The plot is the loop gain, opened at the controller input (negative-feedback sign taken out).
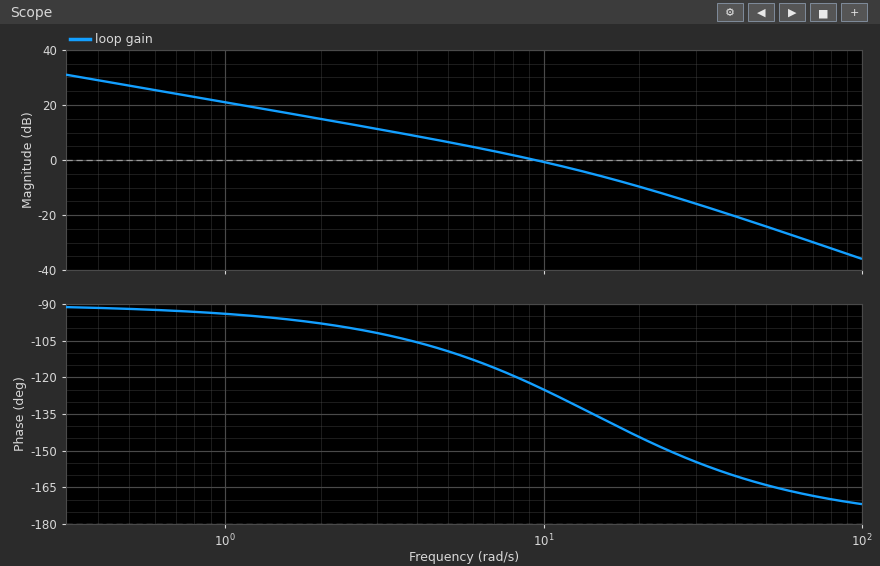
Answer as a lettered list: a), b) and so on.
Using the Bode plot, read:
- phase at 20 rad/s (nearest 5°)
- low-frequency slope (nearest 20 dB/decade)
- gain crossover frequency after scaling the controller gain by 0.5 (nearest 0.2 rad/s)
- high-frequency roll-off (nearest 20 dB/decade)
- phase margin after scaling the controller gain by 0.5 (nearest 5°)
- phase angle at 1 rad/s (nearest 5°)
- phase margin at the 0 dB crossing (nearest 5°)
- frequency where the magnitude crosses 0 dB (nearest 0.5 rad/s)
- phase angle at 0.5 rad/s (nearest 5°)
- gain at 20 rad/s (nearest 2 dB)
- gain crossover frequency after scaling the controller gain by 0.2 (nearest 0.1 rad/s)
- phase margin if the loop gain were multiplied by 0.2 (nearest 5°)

a) -145°
b) -20 dB/decade
c) 5.2 rad/s
d) -40 dB/decade
e) 70°
f) -95°
g) 55°
h) 9.5 rad/s
i) -90°
j) -10 dB
k) 2.2 rad/s
l) 80°
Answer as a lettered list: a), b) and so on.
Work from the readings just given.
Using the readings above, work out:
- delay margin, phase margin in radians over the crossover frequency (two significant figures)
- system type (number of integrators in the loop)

a) 0.10 s
b) 1
